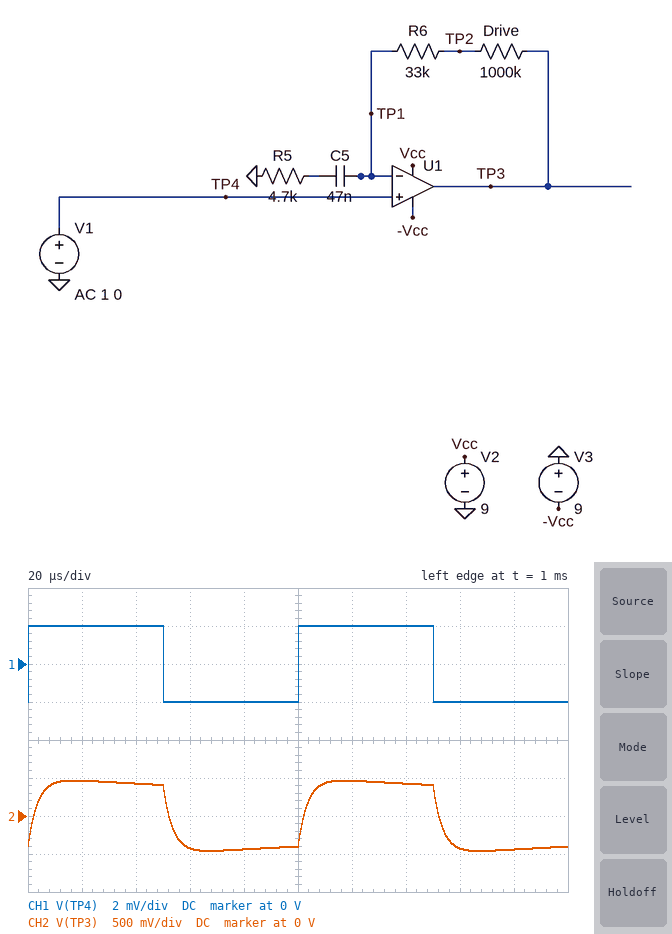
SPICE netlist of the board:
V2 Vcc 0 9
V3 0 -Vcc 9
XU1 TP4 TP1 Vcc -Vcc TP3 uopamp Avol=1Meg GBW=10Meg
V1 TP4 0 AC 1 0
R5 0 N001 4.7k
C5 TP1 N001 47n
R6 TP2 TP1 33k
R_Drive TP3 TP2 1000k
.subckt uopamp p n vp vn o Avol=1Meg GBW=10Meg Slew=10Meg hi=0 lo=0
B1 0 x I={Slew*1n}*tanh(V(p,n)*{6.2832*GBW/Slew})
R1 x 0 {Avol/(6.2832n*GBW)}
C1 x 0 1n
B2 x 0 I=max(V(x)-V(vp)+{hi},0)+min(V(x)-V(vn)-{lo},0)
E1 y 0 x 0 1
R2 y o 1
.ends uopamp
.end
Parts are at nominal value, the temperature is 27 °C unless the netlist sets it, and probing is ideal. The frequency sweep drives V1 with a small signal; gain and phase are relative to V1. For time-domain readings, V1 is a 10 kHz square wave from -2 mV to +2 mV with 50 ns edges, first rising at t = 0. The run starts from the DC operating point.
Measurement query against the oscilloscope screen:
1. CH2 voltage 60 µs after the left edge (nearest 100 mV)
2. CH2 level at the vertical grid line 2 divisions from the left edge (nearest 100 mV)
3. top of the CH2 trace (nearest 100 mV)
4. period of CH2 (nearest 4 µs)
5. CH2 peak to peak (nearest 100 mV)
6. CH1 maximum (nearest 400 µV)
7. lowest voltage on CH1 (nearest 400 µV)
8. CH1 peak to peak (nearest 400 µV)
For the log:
-400 mV
400 mV
500 mV
100 µs
900 mV
2.0 mV
-2.0 mV
4.0 mV
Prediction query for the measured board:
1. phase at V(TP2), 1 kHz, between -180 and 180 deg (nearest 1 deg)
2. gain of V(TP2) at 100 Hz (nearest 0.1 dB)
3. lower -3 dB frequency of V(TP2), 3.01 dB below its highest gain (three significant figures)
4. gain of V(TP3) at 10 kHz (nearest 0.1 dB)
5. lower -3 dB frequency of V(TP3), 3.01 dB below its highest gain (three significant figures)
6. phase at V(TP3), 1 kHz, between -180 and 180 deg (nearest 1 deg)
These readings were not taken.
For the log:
30 deg
3.4 dB
698 Hz
46.8 dB
709 Hz
35 deg
